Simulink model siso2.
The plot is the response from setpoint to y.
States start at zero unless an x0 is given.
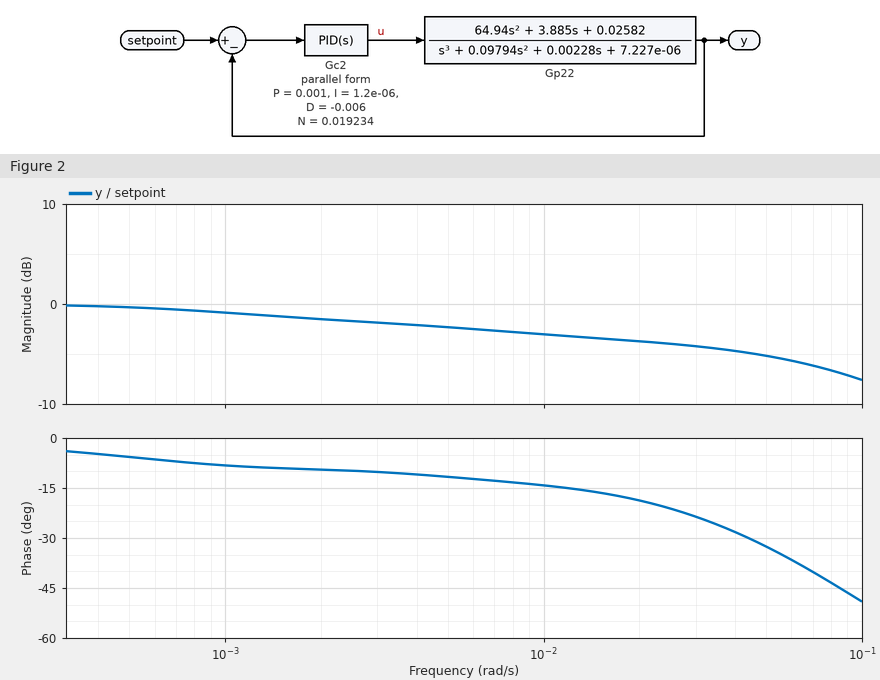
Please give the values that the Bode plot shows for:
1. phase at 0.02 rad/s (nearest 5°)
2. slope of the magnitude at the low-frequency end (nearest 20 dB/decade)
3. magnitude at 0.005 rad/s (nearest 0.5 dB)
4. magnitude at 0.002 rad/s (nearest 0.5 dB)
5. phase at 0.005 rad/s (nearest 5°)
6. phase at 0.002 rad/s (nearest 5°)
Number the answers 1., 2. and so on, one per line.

1. -20°
2. 0 dB/decade
3. -2.5 dB
4. -1.5 dB
5. -10°
6. -10°
